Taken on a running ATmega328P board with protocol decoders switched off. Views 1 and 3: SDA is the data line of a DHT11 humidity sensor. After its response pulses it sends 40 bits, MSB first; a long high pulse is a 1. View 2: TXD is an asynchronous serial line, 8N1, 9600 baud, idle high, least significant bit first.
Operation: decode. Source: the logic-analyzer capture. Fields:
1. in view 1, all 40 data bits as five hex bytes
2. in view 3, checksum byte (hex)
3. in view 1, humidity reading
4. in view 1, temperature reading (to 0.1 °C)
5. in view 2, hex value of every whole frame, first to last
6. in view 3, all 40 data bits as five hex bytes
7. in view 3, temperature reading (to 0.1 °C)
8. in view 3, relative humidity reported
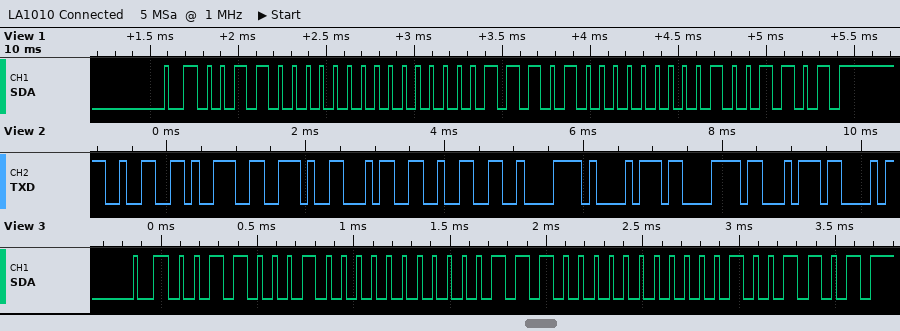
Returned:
30 00 1D 00 4D
0x4D
48 %
29.0 °C
32 39 2E 34 32 C2 A1 C3 A3 43
31 00 1C 00 4D
28.0 °C
49 %
